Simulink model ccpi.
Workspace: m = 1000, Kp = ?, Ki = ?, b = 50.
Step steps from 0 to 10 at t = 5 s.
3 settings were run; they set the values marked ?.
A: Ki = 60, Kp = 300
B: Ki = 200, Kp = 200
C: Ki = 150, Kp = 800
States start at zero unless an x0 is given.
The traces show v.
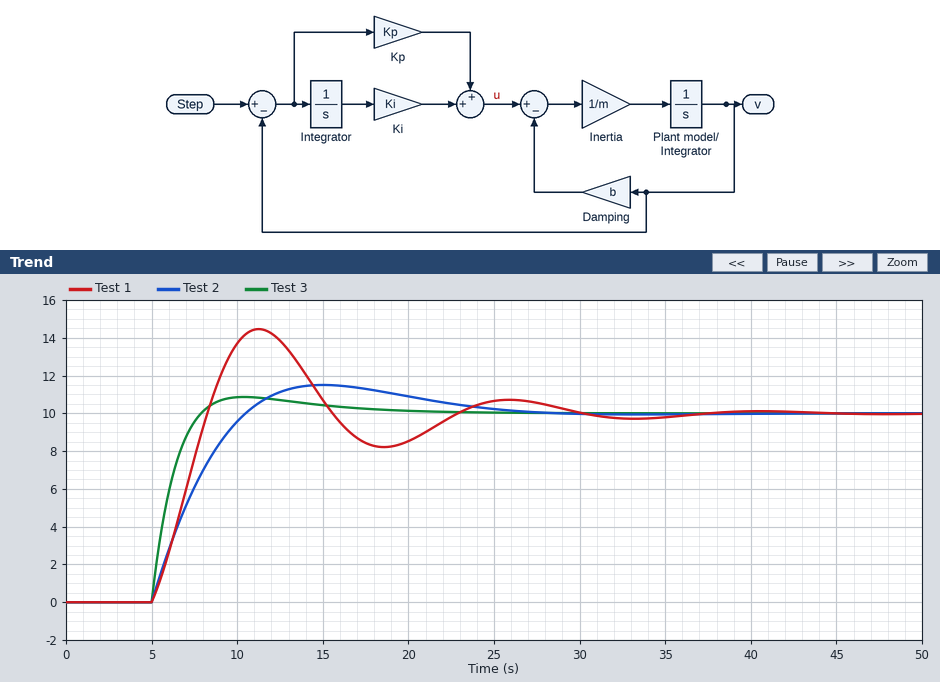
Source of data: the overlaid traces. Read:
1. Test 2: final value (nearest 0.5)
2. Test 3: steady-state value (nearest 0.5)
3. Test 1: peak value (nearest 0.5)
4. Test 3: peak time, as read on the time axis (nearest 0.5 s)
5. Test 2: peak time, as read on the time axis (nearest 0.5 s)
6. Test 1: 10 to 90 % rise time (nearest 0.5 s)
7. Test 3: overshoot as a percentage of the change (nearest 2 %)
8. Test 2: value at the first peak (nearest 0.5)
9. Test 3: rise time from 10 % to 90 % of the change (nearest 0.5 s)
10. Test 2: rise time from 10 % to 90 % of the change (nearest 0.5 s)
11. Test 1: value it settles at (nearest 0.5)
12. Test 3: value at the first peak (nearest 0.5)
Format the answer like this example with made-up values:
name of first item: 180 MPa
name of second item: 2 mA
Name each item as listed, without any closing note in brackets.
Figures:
Test 2: final value: 10.0
Test 3: steady-state value: 10.0
Test 1: peak value: 14.5
Test 3: peak time, as read on the time axis: 10.5 s
Test 2: peak time, as read on the time axis: 15.0 s
Test 1: 10 to 90 % rise time: 2.5 s
Test 3: overshoot as a percentage of the change: 8 %
Test 2: value at the first peak: 11.5
Test 3: rise time from 10 % to 90 % of the change: 2.0 s
Test 2: rise time from 10 % to 90 % of the change: 4.0 s
Test 1: value it settles at: 10.0
Test 3: value at the first peak: 11.0
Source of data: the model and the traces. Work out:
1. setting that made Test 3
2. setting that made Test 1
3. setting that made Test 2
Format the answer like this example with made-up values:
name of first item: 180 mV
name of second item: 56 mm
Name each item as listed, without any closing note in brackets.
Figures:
setting that made Test 3: C
setting that made Test 1: B
setting that made Test 2: A
